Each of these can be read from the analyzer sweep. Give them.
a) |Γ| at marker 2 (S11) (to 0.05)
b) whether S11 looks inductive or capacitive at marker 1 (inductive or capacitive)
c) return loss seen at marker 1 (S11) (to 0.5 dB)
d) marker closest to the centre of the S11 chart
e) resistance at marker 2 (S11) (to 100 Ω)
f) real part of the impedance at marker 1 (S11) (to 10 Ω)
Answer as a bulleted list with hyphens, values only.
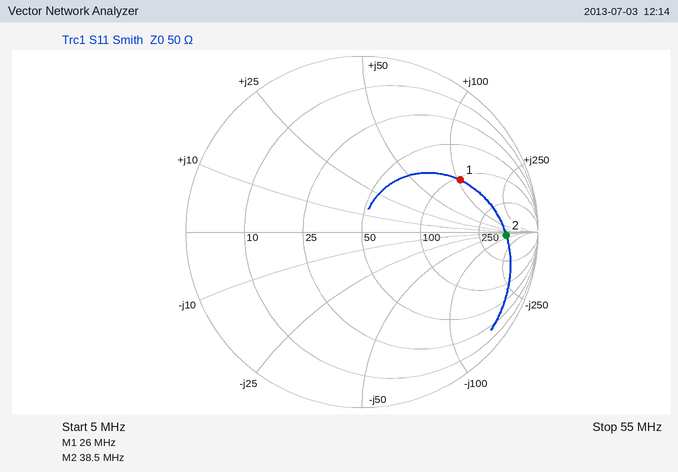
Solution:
- 0.80
- inductive
- 4.0 dB
- marker 1
- 500 Ω
- 110 Ω
